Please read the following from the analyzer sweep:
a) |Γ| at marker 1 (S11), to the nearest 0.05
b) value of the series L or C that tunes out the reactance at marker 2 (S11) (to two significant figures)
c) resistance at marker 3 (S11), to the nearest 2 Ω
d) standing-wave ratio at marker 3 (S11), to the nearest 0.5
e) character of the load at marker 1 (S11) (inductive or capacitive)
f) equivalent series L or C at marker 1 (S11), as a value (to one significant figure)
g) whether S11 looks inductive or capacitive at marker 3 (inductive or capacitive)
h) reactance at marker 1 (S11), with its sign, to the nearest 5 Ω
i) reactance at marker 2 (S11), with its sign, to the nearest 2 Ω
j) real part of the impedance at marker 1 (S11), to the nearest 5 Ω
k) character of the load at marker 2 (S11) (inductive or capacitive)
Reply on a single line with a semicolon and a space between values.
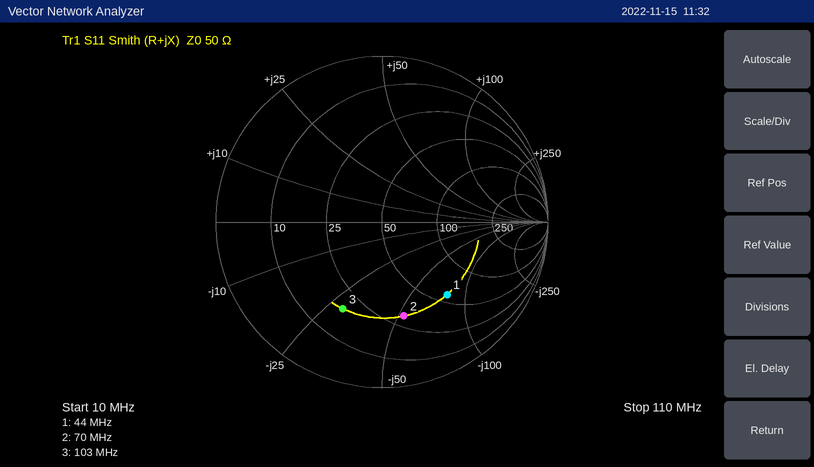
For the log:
0.60; 120 nH; 18 Ω; 3.5; capacitive; 50 pF; capacitive; -80 Ω; -52 Ω; 60 Ω; capacitive
